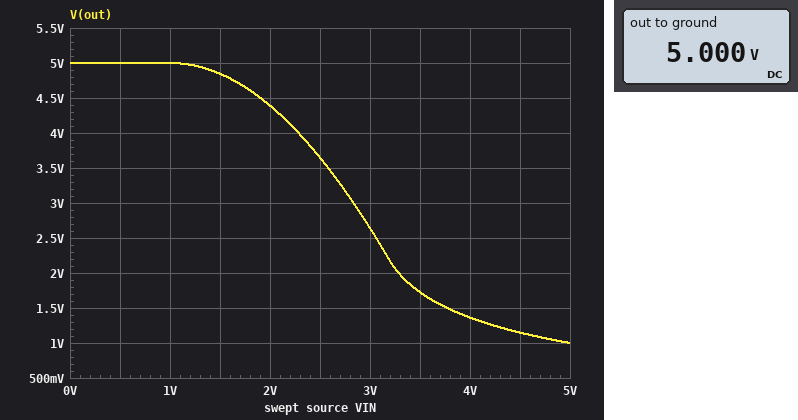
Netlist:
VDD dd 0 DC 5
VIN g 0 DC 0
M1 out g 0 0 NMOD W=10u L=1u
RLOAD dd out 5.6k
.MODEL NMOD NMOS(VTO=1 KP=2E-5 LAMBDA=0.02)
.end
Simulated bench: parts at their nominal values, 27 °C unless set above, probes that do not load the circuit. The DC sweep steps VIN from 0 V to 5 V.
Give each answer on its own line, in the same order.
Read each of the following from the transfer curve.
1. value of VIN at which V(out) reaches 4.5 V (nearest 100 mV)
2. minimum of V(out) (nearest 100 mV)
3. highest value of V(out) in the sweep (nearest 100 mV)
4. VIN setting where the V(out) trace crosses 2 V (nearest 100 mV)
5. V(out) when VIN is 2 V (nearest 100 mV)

1.9 V
1.0 V
5.0 V
3.3 V
4.4 V
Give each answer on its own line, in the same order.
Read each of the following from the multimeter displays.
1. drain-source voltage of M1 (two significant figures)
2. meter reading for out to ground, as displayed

5.0 V
5.000 V
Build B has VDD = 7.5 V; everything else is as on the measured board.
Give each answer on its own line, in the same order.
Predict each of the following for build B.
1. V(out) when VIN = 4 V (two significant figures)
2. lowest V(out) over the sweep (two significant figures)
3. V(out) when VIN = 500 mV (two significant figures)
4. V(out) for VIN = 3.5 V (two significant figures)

2.4 V
1.6 V
7.5 V
3.7 V
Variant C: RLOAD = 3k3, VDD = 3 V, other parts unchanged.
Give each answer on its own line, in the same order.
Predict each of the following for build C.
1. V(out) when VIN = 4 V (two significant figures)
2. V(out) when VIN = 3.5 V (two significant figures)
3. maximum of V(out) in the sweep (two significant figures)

1.1 V
1.3 V
3.0 V
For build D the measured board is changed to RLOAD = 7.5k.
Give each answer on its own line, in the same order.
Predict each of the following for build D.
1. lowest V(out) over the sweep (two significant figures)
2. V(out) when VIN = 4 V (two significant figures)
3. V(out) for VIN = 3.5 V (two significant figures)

770 mV
1.0 V
1.3 V
